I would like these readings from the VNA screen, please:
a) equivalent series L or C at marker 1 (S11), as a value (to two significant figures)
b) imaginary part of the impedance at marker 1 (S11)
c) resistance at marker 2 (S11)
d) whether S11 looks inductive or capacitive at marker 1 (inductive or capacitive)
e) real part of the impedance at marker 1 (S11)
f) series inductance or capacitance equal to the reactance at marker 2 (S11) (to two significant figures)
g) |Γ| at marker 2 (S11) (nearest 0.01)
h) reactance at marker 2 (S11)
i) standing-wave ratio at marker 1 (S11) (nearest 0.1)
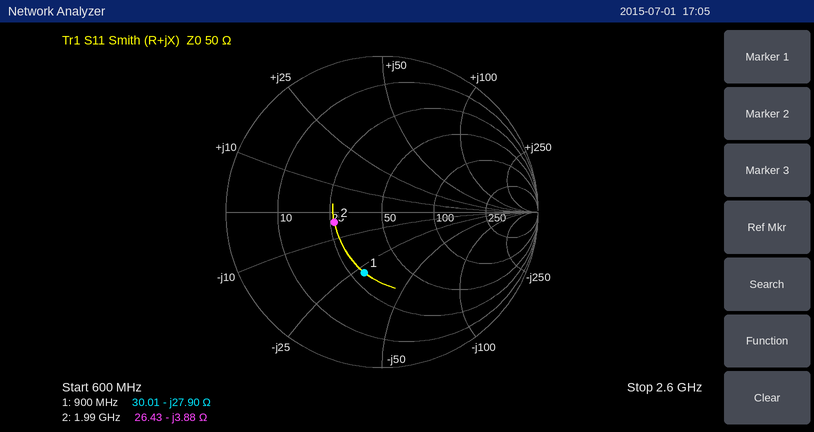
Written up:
6.3 pF
-27.90 Ω
26.43 Ω
capacitive
30.01 Ω
21 pF
0.31
-3.88 Ω
2.4
